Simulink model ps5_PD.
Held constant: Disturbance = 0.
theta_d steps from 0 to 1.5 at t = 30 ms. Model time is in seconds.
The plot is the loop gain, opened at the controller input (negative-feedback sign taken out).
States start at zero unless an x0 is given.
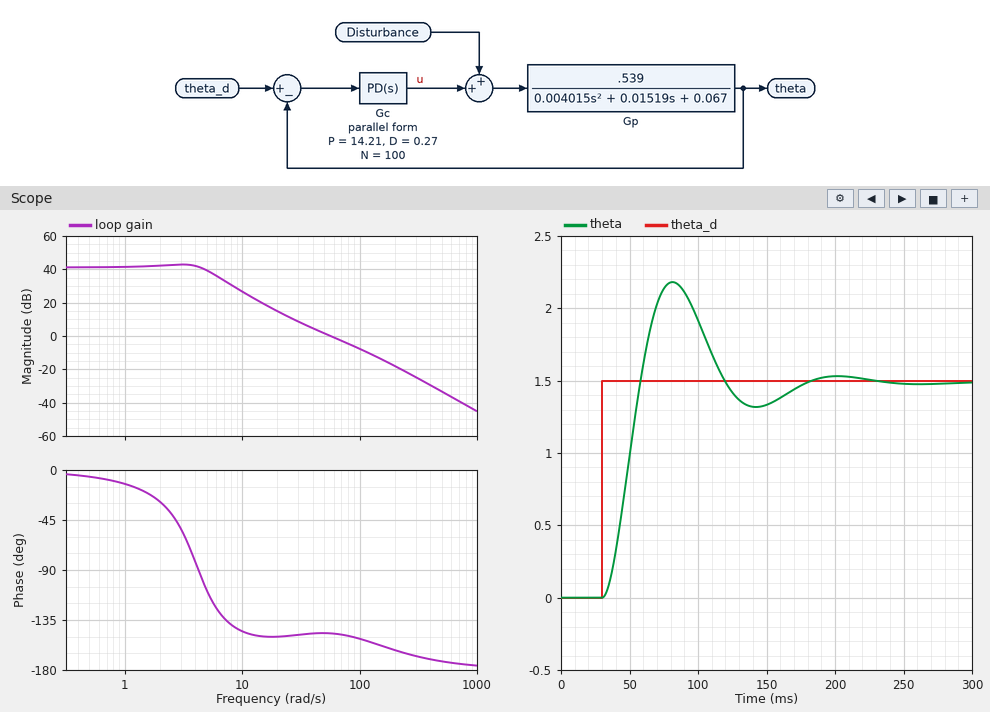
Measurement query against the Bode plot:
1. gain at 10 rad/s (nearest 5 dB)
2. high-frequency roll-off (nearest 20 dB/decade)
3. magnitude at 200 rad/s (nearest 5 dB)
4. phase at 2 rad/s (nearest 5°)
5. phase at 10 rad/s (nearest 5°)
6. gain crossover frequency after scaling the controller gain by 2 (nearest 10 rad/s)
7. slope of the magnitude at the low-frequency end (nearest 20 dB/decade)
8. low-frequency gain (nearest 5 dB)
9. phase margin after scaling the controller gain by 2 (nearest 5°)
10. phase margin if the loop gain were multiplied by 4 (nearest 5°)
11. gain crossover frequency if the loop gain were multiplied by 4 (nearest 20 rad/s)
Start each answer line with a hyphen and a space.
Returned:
- 25 dB
- -40 dB/decade
- -20 dB
- -30°
- -145°
- 90 rad/s
- 0 dB/decade
- 40 dB
- 30°
- 25°
- 140 rad/s
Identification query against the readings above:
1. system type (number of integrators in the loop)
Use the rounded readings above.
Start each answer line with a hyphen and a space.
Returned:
- 0
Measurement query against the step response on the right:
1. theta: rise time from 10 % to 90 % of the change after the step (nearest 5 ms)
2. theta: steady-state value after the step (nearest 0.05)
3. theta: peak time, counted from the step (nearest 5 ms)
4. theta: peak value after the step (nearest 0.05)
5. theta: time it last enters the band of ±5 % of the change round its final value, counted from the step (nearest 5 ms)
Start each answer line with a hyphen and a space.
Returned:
- 20 ms
- 1.50
- 50 ms
- 2.20
- 135 ms
